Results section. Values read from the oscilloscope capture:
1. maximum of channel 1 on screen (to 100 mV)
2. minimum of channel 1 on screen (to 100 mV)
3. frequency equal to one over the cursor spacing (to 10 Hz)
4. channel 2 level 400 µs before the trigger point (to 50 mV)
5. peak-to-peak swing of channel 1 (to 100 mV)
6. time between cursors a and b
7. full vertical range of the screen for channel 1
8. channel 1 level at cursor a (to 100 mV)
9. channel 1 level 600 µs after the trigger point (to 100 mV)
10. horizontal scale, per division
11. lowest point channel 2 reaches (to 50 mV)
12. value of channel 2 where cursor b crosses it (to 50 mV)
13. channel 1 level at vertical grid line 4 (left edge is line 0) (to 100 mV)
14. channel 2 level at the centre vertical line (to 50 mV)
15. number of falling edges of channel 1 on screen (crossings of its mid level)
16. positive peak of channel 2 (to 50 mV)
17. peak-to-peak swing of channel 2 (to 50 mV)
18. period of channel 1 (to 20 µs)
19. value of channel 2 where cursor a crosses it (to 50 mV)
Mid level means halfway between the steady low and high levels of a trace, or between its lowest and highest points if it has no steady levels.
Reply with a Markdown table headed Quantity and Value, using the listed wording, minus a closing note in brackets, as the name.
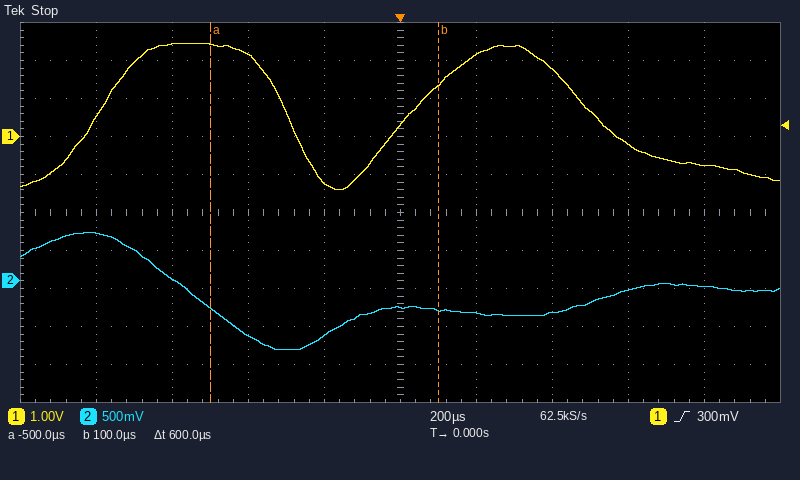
| Quantity | Value |
|---|---|
| maximum of channel 1 on screen | 2.4 V |
| minimum of channel 1 on screen | -1.4 V |
| frequency equal to one over the cursor spacing | 1.67 kHz |
| channel 2 level 400 µs before the trigger point | -700 mV |
| peak-to-peak swing of channel 1 | 3.8 V |
| time between cursors a and b | 600 µs |
| full vertical range of the screen for channel 1 | 10 V |
| channel 1 level at cursor a | 2.4 V |
| channel 1 level 600 µs after the trigger point | -200 mV |
| horizontal scale, per division | 200 µs |
| lowest point channel 2 reaches | -900 mV |
| value of channel 2 where cursor b crosses it | -400 mV |
| channel 1 level at vertical grid line 4 (left edge is line 0) | -1.2 V |
| channel 2 level at the centre vertical line | -350 mV |
| number of falling edges of channel 1 on screen | 2 |
| positive peak of channel 2 | 650 mV |
| peak-to-peak swing of channel 2 | 1.55 V |
| period of channel 1 | 820 µs |
| value of channel 2 where cursor a crosses it | -350 mV |
